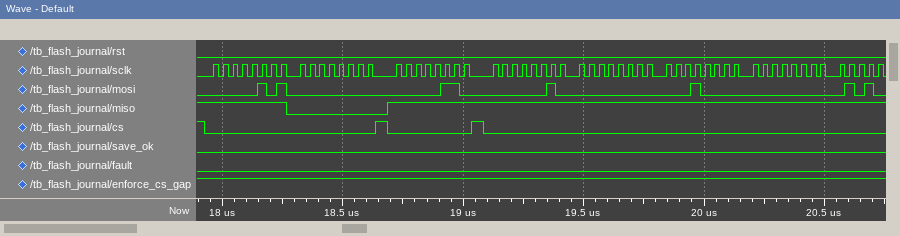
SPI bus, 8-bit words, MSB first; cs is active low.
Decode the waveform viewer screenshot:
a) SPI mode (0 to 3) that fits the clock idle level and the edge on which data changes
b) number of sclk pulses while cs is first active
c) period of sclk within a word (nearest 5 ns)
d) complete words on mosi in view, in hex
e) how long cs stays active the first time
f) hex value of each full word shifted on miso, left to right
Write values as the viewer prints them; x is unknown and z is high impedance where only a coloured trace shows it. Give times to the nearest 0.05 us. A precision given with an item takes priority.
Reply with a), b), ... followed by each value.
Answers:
a) 0
b) 16
c) 40 ns
d) 05, 00, 06, 02, 00, 10, 00
e) 0.7 us
f) FF, 00, FF, FF, FF, FF, FF
